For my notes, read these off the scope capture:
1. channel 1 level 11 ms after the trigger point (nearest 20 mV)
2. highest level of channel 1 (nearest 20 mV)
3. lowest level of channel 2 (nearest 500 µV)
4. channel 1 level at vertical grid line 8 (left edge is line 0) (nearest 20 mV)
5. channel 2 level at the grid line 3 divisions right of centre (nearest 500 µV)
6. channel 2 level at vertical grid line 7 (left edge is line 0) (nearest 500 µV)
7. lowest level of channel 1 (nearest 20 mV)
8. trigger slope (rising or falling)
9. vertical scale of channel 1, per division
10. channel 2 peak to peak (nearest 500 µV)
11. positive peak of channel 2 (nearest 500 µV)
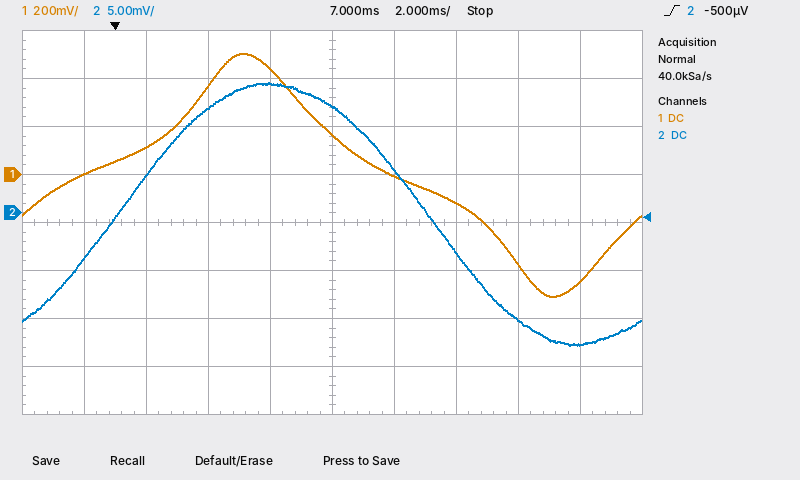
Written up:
-120 mV
500 mV
-14.0 mV
-380 mV
-11.0 mV
-4.0 mV
-500 mV
rising
200 mV
27.5 mV
13.5 mV
